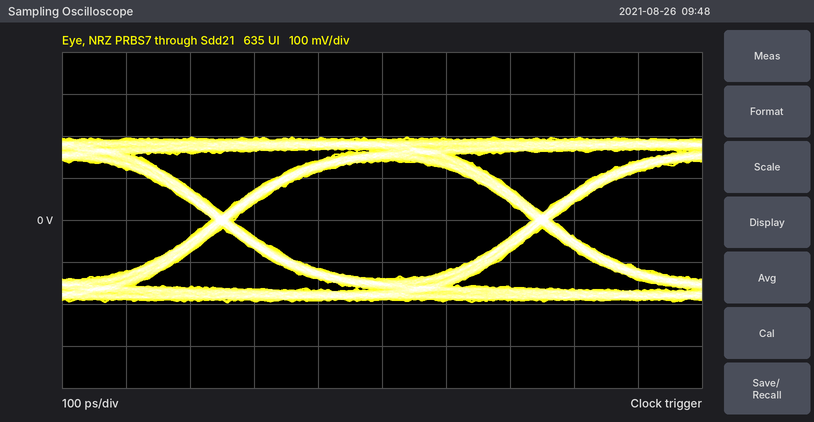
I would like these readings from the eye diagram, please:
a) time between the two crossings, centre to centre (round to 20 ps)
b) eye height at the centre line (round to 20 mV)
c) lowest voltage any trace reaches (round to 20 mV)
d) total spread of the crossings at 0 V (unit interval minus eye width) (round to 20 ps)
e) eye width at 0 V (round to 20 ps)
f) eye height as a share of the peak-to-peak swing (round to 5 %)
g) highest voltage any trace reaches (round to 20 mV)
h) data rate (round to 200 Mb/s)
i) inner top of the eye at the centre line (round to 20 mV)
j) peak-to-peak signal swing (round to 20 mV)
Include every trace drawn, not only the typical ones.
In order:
500 ps
280 mV
-200 mV
40 ps
460 ps
70 %
200 mV
2.0 Gb/s
140 mV
400 mV
